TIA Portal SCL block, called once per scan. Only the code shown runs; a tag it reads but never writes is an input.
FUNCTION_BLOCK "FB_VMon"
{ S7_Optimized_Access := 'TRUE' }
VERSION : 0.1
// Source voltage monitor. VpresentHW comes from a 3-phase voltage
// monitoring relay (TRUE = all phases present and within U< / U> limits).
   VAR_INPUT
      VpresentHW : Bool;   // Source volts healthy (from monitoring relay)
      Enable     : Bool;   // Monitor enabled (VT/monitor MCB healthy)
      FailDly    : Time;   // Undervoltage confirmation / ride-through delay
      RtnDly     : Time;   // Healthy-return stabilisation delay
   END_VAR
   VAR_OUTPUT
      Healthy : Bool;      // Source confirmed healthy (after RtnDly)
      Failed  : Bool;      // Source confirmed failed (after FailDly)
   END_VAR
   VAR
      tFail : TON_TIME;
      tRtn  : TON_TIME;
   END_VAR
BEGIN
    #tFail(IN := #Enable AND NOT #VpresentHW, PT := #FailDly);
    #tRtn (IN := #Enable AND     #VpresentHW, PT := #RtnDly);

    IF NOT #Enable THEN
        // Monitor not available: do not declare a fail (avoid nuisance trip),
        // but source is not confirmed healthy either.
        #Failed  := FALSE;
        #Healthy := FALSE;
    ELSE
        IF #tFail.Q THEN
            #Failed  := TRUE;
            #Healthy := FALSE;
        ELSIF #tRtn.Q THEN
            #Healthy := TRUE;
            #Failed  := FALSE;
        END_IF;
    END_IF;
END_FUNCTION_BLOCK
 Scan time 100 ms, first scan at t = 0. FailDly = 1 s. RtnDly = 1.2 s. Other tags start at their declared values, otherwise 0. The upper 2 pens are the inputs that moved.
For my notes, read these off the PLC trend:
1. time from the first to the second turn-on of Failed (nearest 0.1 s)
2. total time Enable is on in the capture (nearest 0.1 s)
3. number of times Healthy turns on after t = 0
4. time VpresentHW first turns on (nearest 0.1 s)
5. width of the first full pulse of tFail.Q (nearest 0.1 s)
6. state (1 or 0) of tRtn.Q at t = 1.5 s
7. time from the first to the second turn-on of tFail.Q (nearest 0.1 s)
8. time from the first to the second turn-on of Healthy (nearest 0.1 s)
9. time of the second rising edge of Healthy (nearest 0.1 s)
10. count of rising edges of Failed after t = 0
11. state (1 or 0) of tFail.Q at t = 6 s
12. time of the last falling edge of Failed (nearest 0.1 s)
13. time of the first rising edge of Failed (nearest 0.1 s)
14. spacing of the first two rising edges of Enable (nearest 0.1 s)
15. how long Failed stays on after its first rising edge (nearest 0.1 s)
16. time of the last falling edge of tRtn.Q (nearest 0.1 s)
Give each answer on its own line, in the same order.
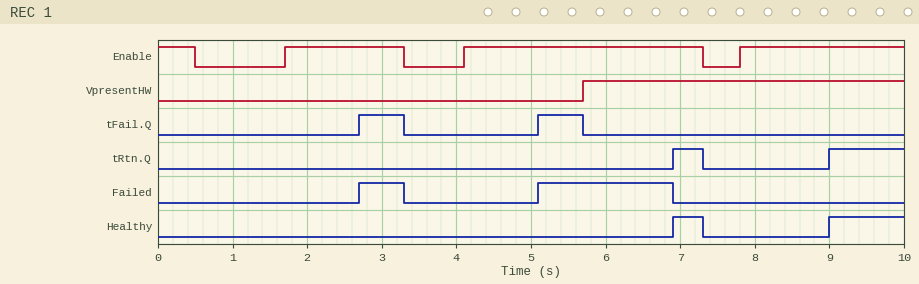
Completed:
2.4 s
7.5 s
2
5.7 s
0.6 s
0
2.4 s
2.1 s
9.0 s
2
0
6.9 s
2.7 s
2.4 s
0.6 s
7.3 s
